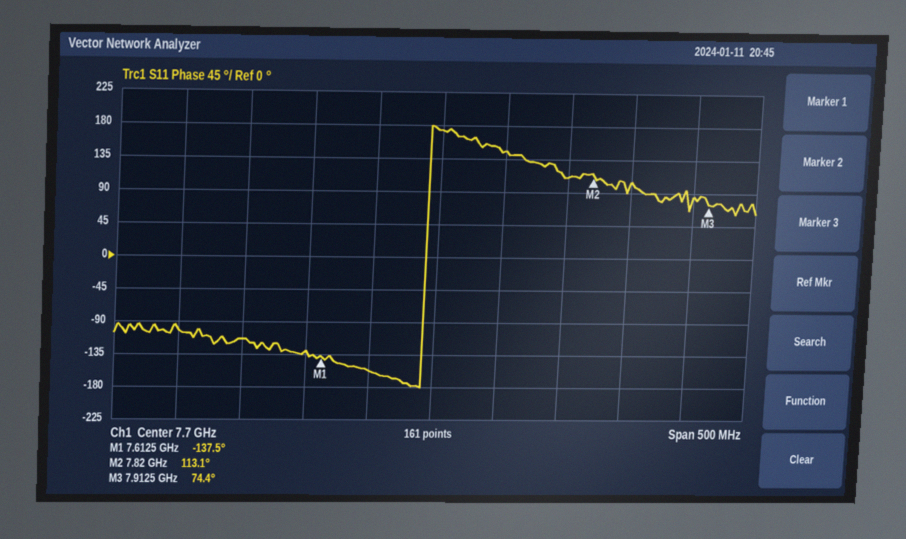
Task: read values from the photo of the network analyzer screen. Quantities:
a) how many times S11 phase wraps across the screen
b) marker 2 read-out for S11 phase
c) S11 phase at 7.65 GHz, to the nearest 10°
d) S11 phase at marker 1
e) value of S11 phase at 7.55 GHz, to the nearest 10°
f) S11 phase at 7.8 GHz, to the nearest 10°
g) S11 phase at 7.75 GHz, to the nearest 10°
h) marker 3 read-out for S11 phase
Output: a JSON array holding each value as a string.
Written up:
["1", "113.1°", "-160°", "-137.5°", "-110°", "110°", "150°", "74.4°"]
